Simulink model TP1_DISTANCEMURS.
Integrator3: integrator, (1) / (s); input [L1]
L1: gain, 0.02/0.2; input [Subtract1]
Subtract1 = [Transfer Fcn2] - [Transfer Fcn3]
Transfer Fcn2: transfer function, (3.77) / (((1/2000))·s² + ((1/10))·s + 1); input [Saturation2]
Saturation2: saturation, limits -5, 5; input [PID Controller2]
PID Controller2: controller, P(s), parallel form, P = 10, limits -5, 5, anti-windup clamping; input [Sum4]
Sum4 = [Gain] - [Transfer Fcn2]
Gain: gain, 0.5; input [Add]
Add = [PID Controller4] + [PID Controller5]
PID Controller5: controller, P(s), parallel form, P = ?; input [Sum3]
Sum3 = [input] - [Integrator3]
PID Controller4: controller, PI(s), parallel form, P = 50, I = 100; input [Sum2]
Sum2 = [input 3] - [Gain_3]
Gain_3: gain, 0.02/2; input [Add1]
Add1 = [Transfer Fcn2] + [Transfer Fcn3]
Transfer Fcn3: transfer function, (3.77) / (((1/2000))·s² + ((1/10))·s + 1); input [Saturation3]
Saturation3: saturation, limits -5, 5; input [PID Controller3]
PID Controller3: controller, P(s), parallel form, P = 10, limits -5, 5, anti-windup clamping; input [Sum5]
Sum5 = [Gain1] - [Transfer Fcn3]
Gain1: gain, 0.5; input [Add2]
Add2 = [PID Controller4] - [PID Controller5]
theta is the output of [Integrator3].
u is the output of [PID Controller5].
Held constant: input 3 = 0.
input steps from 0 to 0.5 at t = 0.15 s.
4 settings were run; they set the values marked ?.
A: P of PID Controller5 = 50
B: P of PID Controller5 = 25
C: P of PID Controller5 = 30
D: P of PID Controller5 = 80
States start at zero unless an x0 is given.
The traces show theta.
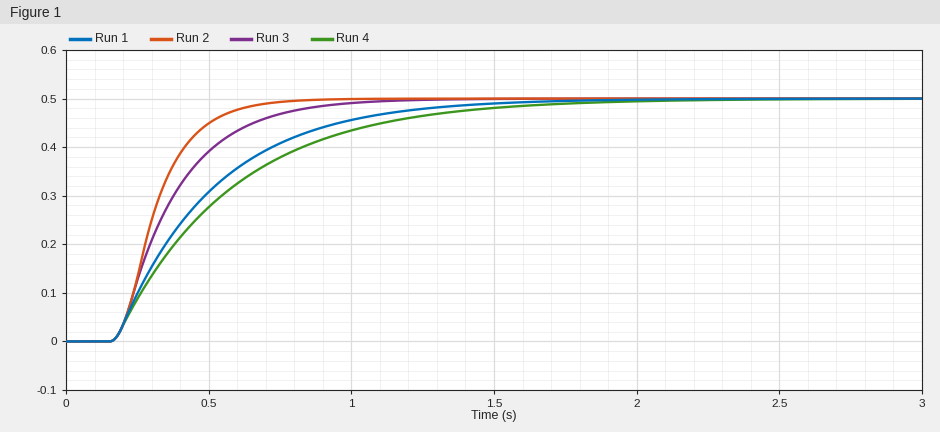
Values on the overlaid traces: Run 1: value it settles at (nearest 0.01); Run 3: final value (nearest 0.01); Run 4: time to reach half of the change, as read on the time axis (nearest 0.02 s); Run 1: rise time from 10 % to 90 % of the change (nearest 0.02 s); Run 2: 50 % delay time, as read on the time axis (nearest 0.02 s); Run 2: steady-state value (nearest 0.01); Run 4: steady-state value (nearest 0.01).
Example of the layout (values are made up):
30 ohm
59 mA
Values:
0.50
0.50
0.46 s
0.74 s
0.30 s
0.50
0.50
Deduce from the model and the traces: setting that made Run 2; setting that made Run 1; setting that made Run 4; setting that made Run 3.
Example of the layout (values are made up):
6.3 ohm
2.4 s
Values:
D
C
B
A
